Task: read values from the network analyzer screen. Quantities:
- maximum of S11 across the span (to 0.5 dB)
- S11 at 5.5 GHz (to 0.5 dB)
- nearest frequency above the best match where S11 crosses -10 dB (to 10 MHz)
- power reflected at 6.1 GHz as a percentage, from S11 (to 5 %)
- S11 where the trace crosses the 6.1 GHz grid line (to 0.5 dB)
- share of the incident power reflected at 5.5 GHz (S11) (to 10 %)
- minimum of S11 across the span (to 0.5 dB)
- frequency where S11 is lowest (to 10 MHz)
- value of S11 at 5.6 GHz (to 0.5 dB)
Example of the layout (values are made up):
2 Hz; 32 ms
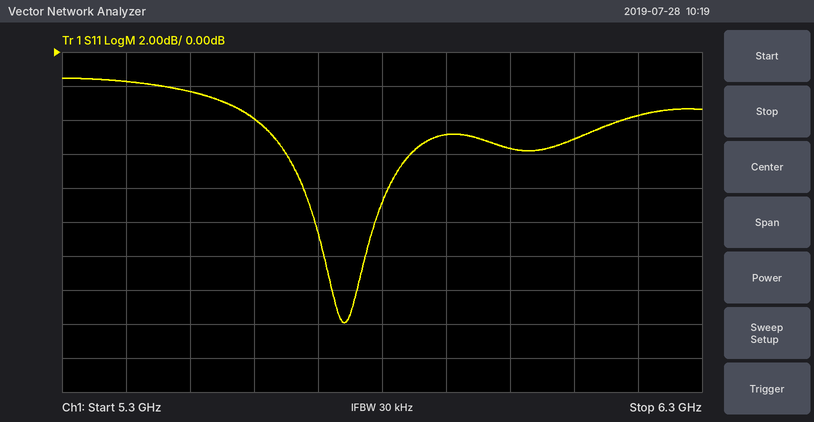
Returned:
-1.5 dB; -2.5 dB; 5.79 GHz; 30 %; -5.0 dB; 60 %; -16.0 dB; 5.74 GHz; -4.0 dB
